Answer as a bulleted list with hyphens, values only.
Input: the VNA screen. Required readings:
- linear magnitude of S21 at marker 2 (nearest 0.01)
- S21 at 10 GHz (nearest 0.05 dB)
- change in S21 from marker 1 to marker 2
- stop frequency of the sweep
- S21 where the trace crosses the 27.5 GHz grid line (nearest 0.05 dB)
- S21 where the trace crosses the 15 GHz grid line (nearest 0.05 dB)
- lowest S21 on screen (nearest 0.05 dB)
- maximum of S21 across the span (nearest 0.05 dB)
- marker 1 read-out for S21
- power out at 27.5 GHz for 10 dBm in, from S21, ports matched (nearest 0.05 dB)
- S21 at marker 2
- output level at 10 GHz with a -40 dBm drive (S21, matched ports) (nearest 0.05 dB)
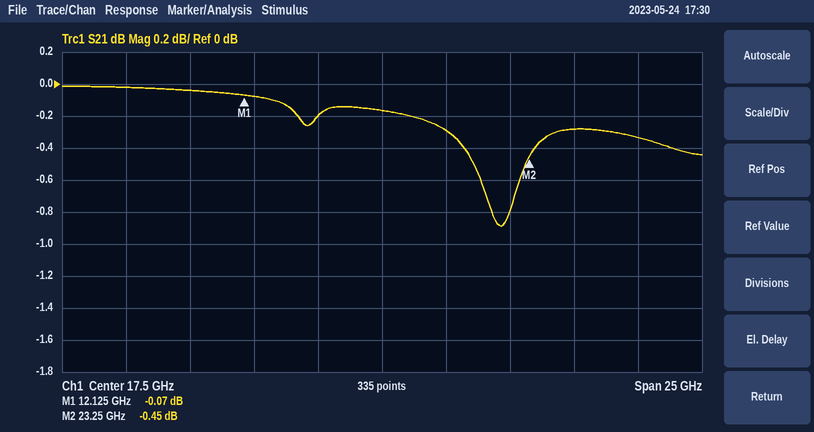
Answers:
- 0.95
- -0.05 dB
- -0.38 dB
- 30 GHz
- -0.35 dB
- -0.20 dB
- -0.90 dB
- 0.00 dB
- -0.07 dB
- 9.65 dBm
- -0.45 dB
- -40.05 dBm
